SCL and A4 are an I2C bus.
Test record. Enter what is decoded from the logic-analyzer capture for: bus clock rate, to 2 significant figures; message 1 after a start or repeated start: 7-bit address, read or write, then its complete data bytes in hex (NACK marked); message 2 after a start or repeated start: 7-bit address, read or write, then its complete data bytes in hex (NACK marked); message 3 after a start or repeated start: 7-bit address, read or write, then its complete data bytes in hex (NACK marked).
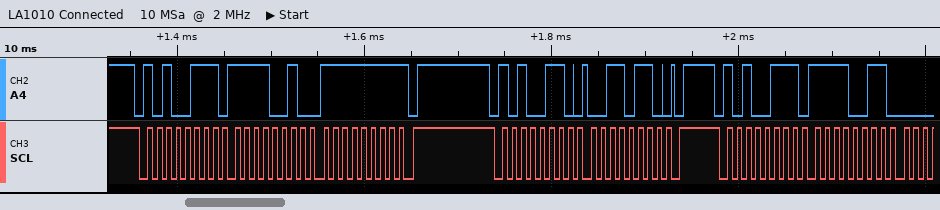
100 kHz
0x53 read: F2 FF NACK
0x53 write: 36
0x53 read: F3
